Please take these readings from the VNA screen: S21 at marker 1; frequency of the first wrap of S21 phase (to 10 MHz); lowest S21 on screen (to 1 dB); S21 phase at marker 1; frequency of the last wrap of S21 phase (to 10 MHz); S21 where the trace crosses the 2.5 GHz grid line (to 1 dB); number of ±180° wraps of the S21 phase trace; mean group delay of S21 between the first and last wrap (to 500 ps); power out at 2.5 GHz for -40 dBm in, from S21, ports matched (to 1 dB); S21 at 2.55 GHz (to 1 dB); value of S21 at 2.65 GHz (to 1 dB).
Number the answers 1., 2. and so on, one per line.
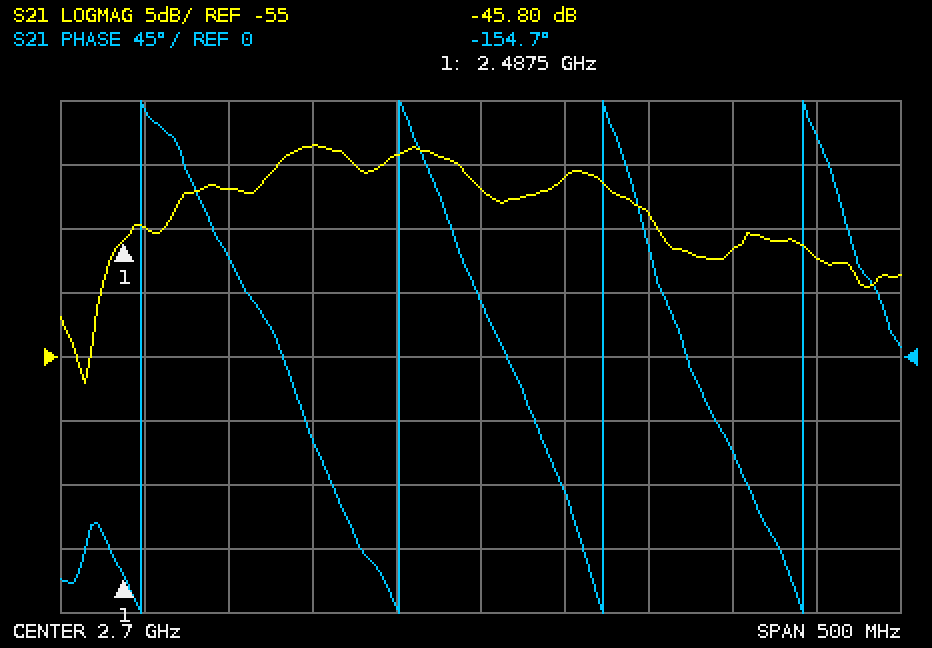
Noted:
1. -45.80 dB
2. 2.50 GHz
3. -57 dB
4. -154.7°
5. 2.89 GHz
6. -45 dB
7. 4
8. 7.5 ns
9. -85 dBm
10. -42 dB
11. -39 dB
